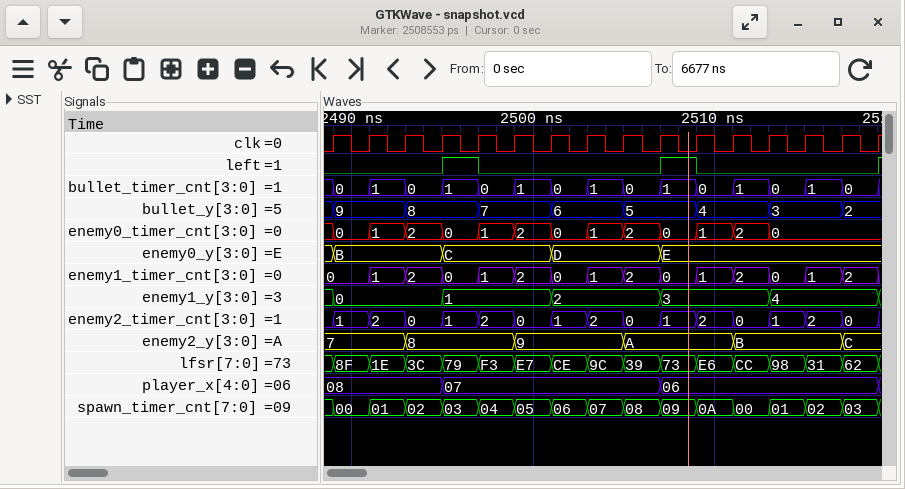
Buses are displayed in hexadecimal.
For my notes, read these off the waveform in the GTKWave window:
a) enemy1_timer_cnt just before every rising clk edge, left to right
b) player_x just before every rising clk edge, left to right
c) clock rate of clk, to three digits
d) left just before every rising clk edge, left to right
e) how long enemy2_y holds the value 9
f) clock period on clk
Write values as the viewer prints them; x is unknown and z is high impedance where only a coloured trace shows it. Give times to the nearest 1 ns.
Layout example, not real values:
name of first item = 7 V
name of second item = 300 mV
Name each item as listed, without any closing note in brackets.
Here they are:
enemy1_timer_cnt just before every rising clk edge, left to right = 0, 0, 1, 2, 0, 1, 2, 0, 1, 2, 0, 1, 2, 0, 1, 2
player_x just before every rising clk edge, left to right = 08, 08, 08, 08, 07, 07, 07, 07, 07, 07, 06, 06, 06, 06, 06, 06
clock rate of clk, to three digits = 500 MHz
left just before every rising clk edge, left to right = 0 0 0 0 1 0 0 0 0 0 1 0 0 0 0 0
how long enemy2_y holds the value 9 = 6 ns
clock period on clk = 2 ns
